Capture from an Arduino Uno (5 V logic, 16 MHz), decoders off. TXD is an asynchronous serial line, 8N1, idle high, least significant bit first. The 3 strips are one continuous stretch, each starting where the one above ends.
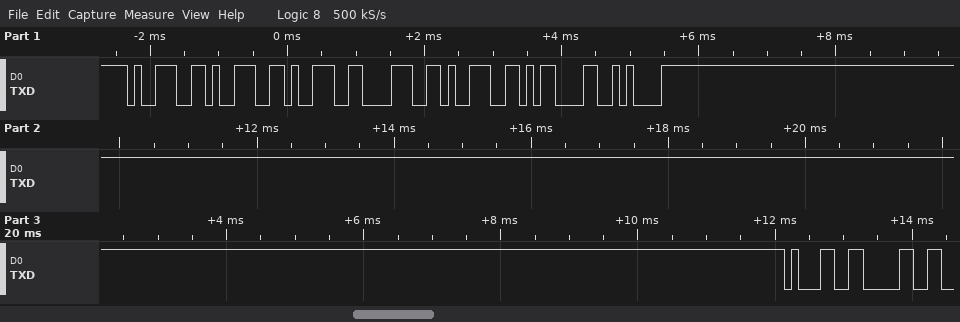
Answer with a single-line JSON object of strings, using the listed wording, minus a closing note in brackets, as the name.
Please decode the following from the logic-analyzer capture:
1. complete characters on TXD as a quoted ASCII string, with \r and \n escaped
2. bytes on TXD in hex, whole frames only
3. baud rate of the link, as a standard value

{"complete characters on TXD as a quoted ASCII string, with \\r and \\n escaped": "\"99989\\r\\n10\"", "bytes on TXD in hex, whole frames only": "0x39 0x39 0x39 0x38 0x39 0x0D 0x0A 0x31 0x30", "baud rate of the link, as a standard value": "9600 baud"}
